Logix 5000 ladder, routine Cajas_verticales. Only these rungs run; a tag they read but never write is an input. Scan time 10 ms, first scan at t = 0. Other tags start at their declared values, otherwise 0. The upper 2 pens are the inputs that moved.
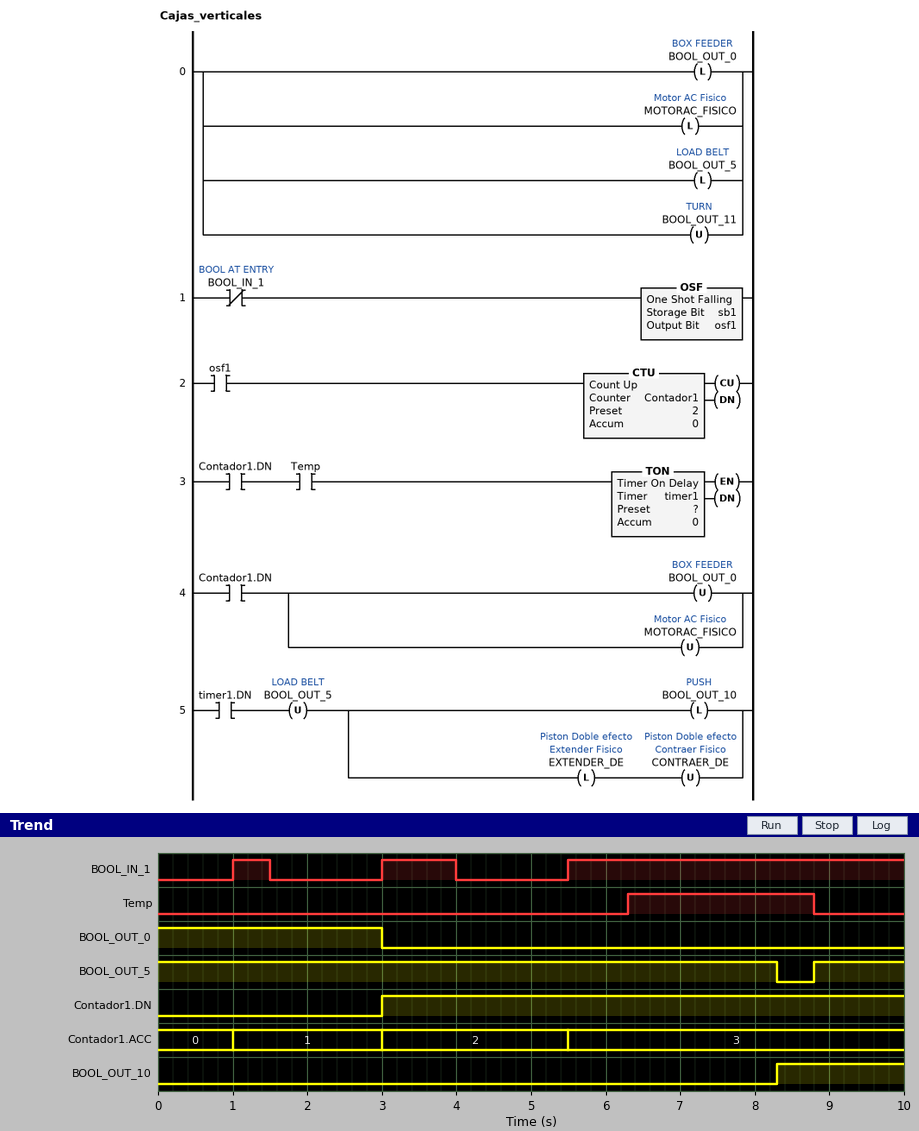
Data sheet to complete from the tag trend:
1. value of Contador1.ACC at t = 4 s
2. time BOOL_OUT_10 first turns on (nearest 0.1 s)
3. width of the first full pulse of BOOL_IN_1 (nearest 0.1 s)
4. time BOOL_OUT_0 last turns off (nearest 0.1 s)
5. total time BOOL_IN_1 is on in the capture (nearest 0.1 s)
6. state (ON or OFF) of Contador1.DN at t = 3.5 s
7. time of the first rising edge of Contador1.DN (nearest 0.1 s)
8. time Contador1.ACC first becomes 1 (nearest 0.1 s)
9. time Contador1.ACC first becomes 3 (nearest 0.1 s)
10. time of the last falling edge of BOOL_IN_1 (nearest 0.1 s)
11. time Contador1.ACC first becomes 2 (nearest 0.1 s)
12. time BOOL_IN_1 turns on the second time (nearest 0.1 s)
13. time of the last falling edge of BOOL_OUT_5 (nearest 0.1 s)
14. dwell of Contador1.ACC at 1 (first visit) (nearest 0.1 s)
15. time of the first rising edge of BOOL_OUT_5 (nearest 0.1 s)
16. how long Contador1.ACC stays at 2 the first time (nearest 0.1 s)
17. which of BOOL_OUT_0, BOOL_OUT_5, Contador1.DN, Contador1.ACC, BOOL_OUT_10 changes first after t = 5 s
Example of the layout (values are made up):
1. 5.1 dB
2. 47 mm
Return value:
1. 2
2. 8.3 s
3. 0.5 s
4. 3.0 s
5. 6.0 s
6. ON
7. 3.0 s
8. 1.0 s
9. 5.5 s
10. 4.0 s
11. 3.0 s
12. 3.0 s
13. 8.3 s
14. 2.0 s
15. 8.8 s
16. 2.5 s
17. Contador1.ACC
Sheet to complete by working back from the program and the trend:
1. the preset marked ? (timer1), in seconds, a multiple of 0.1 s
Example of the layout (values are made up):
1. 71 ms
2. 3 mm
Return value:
1. 2.0 s
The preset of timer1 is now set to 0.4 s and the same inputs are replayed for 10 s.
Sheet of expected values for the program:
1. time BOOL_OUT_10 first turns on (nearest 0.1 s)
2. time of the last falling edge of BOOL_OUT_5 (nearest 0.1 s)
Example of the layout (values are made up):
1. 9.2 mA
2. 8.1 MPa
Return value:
1. 6.7 s
2. 6.7 s
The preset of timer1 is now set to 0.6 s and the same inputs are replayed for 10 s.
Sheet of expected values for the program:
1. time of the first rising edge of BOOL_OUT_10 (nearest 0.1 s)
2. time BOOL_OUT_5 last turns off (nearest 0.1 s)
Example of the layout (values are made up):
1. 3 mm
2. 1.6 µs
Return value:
1. 6.9 s
2. 6.9 s
